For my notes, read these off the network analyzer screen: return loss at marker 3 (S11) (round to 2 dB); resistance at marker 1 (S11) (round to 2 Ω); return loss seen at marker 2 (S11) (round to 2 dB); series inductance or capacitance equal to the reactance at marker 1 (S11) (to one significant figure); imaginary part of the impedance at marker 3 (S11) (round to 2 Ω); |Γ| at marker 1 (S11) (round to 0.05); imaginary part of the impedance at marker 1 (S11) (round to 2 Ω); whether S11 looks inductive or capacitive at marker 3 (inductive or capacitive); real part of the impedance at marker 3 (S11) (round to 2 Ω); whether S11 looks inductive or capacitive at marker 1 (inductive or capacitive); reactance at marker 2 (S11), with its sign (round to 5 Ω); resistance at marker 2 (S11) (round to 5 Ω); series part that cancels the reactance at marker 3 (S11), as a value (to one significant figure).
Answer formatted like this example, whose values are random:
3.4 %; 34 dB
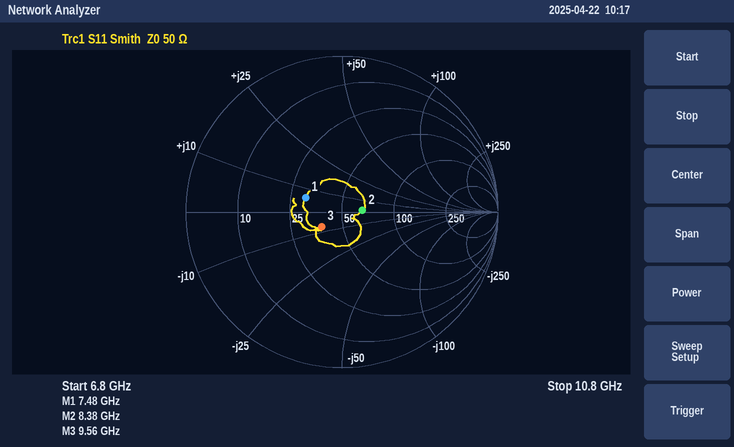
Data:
16 dB; 30 Ω; 18 dB; 100 pH; -8 Ω; 0.25; +6 Ω; capacitive; 38 Ω; inductive; 0 Ω; 65 Ω; 100 pH
